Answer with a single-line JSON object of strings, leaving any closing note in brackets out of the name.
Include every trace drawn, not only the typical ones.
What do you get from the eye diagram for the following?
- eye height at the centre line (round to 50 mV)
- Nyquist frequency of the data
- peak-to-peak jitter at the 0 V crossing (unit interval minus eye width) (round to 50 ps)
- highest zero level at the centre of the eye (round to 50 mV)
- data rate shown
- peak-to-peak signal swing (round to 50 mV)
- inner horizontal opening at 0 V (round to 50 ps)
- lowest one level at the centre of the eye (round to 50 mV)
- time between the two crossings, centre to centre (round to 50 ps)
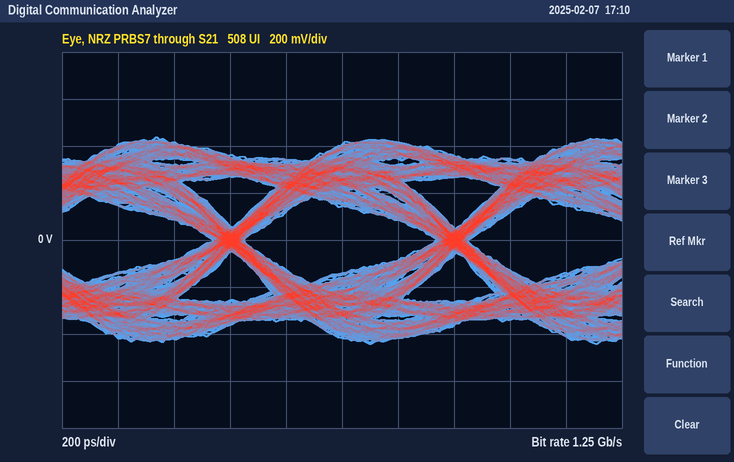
{"eye height at the centre line": "300 mV", "Nyquist frequency of the data": "625 MHz", "peak-to-peak jitter at the 0 V crossing (unit interval minus eye width)": "100 ps", "highest zero level at the centre of the eye": "-150 mV", "data rate shown": "1.25 Gb/s", "peak-to-peak signal swing": "900 mV", "inner horizontal opening at 0 V": "700 ps", "lowest one level at the centre of the eye": "150 mV", "time between the two crossings, centre to centre": "800 ps"}
